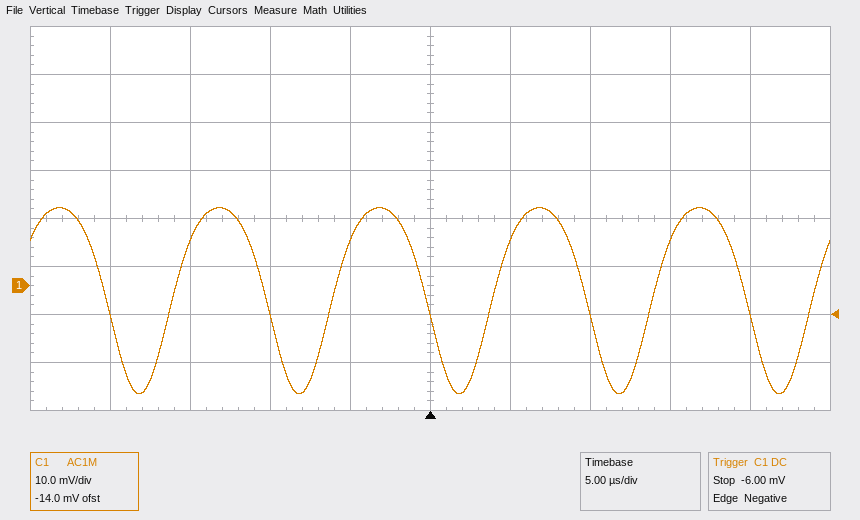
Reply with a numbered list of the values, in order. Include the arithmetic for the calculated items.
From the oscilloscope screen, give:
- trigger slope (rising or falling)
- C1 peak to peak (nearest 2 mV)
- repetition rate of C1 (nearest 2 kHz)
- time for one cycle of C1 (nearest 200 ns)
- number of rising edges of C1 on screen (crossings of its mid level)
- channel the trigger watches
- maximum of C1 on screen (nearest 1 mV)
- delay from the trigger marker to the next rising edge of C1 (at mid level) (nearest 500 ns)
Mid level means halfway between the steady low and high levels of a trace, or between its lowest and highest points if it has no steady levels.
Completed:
1. falling
2. 38 mV
3. 1 / 10.0 µs ≈ 100 kHz
4. 10.0 µs
5. 5
6. C1
7. 16 mV
8. 4.0 µs
